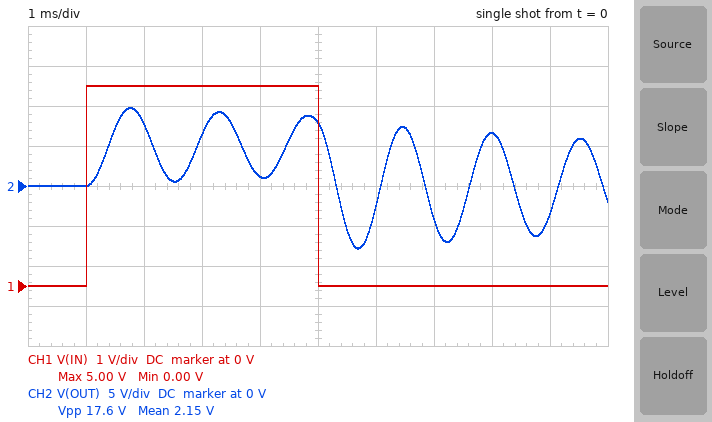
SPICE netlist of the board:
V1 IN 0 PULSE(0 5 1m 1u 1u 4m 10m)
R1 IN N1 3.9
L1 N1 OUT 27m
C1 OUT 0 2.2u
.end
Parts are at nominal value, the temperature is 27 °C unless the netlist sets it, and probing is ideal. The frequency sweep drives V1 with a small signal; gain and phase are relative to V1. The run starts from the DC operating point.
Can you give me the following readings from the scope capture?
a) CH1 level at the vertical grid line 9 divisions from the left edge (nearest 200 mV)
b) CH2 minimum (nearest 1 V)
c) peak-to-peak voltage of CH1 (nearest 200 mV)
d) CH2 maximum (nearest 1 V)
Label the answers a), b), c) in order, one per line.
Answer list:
a) 0 V
b) -8 V
c) 5.0 V
d) 10 V
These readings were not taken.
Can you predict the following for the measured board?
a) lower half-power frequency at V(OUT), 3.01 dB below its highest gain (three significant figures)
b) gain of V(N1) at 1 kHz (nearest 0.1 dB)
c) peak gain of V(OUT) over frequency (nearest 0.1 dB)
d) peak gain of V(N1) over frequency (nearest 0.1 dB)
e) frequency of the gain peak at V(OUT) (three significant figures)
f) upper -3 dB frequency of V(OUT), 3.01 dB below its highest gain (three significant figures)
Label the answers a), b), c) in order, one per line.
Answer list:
a) 641 Hz
b) 0 dB
c) 29.1 dB
d) 0 dB
e) 653 Hz
f) 664 Hz
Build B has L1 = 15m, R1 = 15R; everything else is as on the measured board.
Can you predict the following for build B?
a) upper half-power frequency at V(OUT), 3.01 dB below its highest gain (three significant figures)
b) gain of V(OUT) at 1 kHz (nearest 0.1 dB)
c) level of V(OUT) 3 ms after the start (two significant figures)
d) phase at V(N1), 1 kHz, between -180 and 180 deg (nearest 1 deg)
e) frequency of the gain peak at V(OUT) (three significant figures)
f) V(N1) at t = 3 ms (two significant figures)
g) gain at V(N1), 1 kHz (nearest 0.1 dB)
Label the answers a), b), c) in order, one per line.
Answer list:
a) 945 Hz
b) 8.7 dB
c) 5.2 V
d) 34 deg
e) 869 Hz
f) 5.3 V
g) -1.7 dB
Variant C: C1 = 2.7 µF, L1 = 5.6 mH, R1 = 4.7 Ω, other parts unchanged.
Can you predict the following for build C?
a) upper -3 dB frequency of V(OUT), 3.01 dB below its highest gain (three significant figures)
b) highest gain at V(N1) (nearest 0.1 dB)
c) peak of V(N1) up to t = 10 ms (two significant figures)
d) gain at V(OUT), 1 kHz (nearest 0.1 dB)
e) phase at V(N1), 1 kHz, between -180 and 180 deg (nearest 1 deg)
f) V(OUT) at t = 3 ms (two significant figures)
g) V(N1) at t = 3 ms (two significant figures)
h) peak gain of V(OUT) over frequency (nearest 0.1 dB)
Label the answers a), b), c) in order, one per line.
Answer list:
a) 1.36 kHz
b) 0 dB
c) 5.4 V
d) 7.7 dB
e) -11 deg
f) 6.9 V
g) 5.1 V
h) 19.7 dB
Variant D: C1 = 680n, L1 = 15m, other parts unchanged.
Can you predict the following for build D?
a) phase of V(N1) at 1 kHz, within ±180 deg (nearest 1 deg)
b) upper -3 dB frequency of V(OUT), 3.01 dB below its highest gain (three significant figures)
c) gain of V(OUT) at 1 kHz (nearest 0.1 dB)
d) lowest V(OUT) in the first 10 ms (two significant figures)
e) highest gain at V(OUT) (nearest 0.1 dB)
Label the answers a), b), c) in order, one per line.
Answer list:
a) -2 deg
b) 1.60 kHz
c) 4.5 dB
d) -6.3 V
e) 31.6 dB
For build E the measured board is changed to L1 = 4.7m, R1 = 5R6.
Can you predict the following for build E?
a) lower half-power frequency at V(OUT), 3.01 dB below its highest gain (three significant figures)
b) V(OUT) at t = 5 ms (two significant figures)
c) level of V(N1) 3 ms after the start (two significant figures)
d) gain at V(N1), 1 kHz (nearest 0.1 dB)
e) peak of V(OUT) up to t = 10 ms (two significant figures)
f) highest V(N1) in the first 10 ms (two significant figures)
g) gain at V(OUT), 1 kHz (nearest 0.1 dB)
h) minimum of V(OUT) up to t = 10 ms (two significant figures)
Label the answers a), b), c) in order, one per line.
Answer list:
a) 1.46 kHz
b) 5.0 V
c) 4.9 V
d) -0.1 dB
e) 9.1 V
f) 5.5 V
g) 4.5 dB
h) -4.1 V
